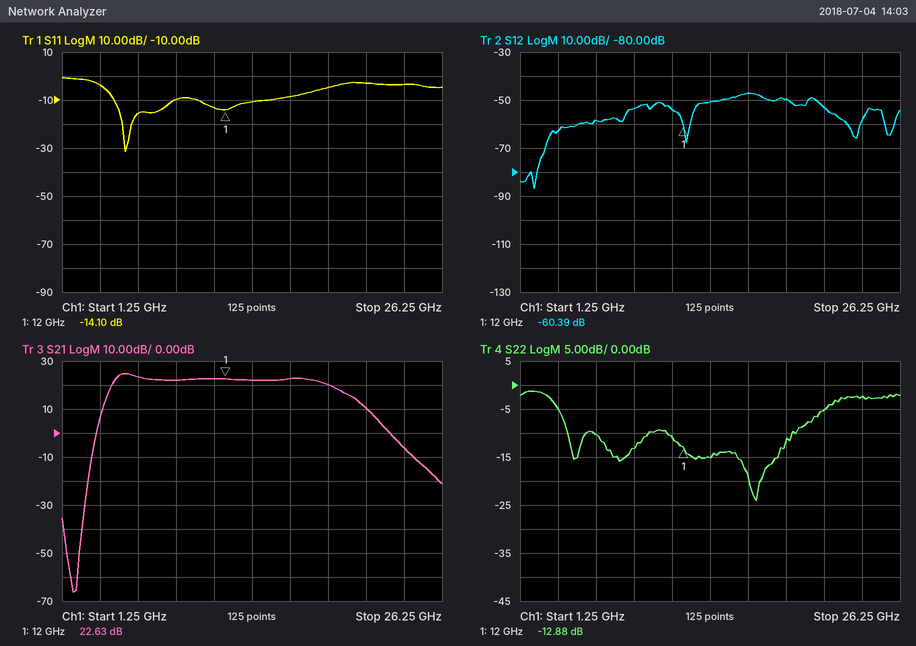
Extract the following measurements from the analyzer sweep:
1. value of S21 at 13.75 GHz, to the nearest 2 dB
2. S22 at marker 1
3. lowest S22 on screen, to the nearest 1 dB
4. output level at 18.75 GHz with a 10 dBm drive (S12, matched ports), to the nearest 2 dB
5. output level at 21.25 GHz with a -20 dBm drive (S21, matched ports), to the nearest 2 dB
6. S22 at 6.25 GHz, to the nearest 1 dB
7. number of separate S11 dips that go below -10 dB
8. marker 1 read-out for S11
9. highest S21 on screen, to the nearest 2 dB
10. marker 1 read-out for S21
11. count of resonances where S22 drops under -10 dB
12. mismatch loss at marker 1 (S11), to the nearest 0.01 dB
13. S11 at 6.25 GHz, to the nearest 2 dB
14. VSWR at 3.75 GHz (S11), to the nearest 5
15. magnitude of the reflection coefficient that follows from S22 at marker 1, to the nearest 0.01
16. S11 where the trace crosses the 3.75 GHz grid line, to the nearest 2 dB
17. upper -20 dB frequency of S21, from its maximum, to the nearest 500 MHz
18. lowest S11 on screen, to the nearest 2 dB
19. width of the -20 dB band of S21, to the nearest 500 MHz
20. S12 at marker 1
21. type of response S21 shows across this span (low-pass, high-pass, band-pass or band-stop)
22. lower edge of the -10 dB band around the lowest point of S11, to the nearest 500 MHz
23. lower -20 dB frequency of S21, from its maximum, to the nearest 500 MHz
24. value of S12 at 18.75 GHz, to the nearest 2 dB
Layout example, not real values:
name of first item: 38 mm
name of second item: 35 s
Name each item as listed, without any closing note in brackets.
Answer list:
value of S21 at 13.75 GHz, to the nearest 2 dB: 22 dB
S22 at marker 1: -12.88 dB
lowest S22 on screen, to the nearest 1 dB: -24 dB
output level at 18.75 GHz with a 10 dBm drive (S12, matched ports), to the nearest 2 dB: -40 dBm
output level at 21.25 GHz with a -20 dBm drive (S21, matched ports), to the nearest 2 dB: -10 dBm
S22 at 6.25 GHz, to the nearest 1 dB: -10 dB
number of separate S11 dips that go below -10 dB: 2
marker 1 read-out for S11: -14.10 dB
highest S21 on screen, to the nearest 2 dB: 24 dB
marker 1 read-out for S21: 22.63 dB
count of resonances where S22 drops under -10 dB: 3
mismatch loss at marker 1 (S11), to the nearest 0.01 dB: 0.17 dB
S11 at 6.25 GHz, to the nearest 2 dB: -16 dB
VSWR at 3.75 GHz (S11), to the nearest 5: 5
magnitude of the reflection coefficient that follows from S22 at marker 1, to the nearest 0.01: 0.23
S11 where the trace crosses the 3.75 GHz grid line, to the nearest 2 dB: -4 dB
upper -20 dB frequency of S21, from its maximum, to the nearest 500 MHz: 22.0 GHz
lowest S11 on screen, to the nearest 2 dB: -32 dB
width of the -20 dB band of S21, to the nearest 500 MHz: 18.5 GHz
S12 at marker 1: -60.39 dB
type of response S21 shows across this span: band-pass
lower edge of the -10 dB band around the lowest point of S11, to the nearest 500 MHz: 4.5 GHz
lower -20 dB frequency of S21, from its maximum, to the nearest 500 MHz: 3.5 GHz
value of S12 at 18.75 GHz, to the nearest 2 dB: -50 dB
